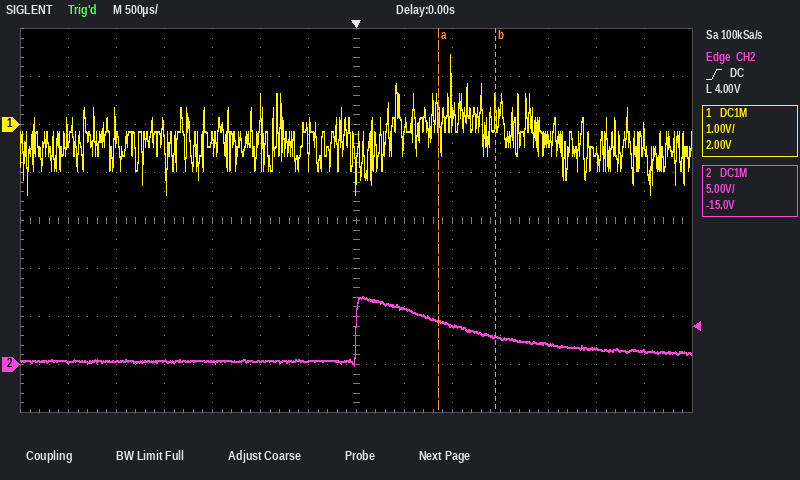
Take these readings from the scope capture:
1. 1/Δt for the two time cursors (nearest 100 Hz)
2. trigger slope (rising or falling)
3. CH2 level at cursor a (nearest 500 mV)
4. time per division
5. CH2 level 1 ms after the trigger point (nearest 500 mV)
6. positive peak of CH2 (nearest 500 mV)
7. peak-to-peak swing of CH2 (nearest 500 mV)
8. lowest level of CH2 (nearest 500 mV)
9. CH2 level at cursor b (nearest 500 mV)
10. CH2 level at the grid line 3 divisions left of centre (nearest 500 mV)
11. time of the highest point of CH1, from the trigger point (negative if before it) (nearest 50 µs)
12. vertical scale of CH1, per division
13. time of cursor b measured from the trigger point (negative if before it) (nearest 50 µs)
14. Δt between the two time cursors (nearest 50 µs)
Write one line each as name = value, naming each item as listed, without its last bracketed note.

1/Δt for the two time cursors = 1.7 kHz
trigger slope = rising
CH2 level at cursor a = 4.5 V
time per division = 500 µs
CH2 level 1 ms after the trigger point = 4.0 V
positive peak of CH2 = 7.0 V
peak-to-peak swing of CH2 = 7.0 V
lowest level of CH2 = 0.0 V
CH2 level at cursor b = 3.0 V
CH2 level at the grid line 3 divisions left of centre = 500 mV
time of the highest point of CH1, from the trigger point (negative if before it) = +1.00 ms
vertical scale of CH1, per division = 1 V
time of cursor b measured from the trigger point (negative if before it) = +1.45 ms
Δt between the two time cursors = 600 µs
